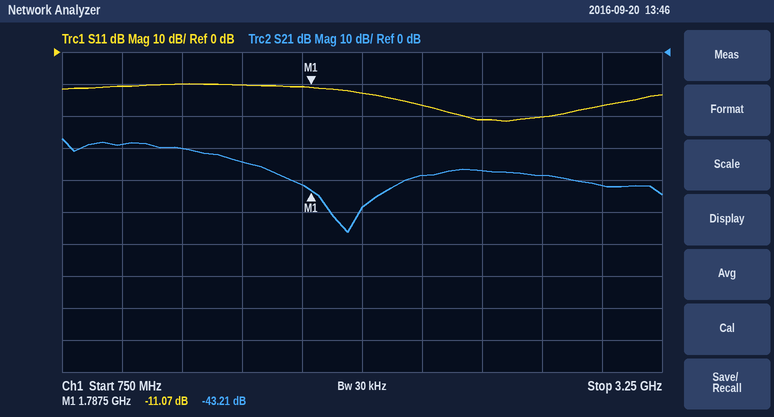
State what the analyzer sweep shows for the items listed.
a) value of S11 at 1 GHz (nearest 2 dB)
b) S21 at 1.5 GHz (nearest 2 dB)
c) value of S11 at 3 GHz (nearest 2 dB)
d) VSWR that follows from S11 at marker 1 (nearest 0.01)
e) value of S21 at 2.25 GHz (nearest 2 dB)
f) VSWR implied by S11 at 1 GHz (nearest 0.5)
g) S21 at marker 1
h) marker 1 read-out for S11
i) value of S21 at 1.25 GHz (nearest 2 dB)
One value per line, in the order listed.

-10 dB
-34 dB
-16 dB
1.78
-38 dB
2.0
-43.21 dB
-11.07 dB
-30 dB
